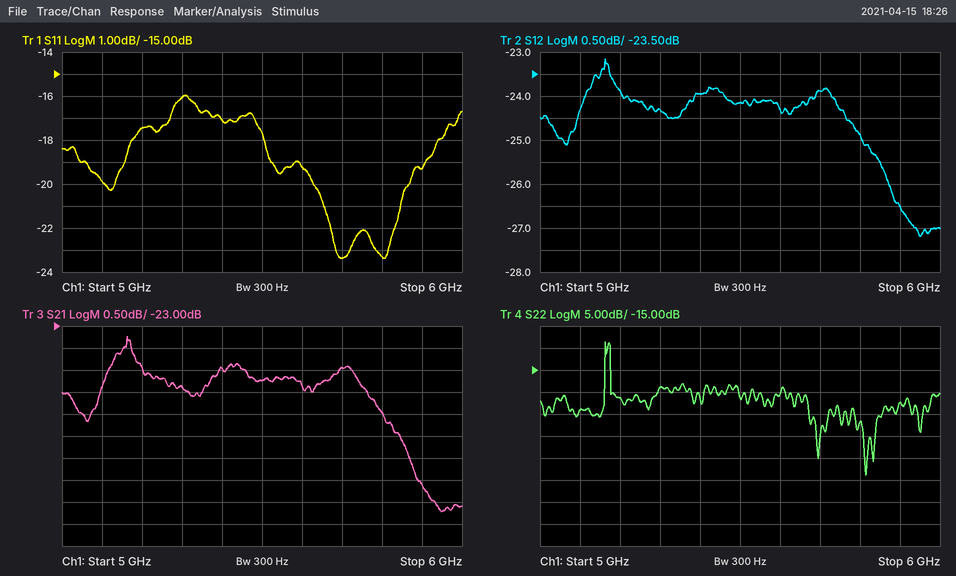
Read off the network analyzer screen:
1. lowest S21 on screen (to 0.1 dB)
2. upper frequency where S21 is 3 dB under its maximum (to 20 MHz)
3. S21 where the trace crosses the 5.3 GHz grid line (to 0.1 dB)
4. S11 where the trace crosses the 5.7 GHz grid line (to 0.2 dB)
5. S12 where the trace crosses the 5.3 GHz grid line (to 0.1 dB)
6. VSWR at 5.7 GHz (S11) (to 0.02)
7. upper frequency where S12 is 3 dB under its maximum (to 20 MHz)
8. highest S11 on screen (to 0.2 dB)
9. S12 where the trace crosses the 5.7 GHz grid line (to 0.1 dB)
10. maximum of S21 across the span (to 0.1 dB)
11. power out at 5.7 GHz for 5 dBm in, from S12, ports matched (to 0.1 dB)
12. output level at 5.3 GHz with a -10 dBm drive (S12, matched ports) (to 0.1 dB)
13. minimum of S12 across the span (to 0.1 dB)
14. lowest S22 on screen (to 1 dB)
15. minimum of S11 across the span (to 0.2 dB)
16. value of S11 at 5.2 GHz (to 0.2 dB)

-27.2 dB
5.88 GHz
-24.4 dB
-23.4 dB
-24.3 dB
1.14
5.88 GHz
-16.0 dB
-23.9 dB
-23.2 dB
-18.9 dBm
-34.3 dBm
-27.2 dB
-39 dB
-23.4 dB
-17.4 dB
